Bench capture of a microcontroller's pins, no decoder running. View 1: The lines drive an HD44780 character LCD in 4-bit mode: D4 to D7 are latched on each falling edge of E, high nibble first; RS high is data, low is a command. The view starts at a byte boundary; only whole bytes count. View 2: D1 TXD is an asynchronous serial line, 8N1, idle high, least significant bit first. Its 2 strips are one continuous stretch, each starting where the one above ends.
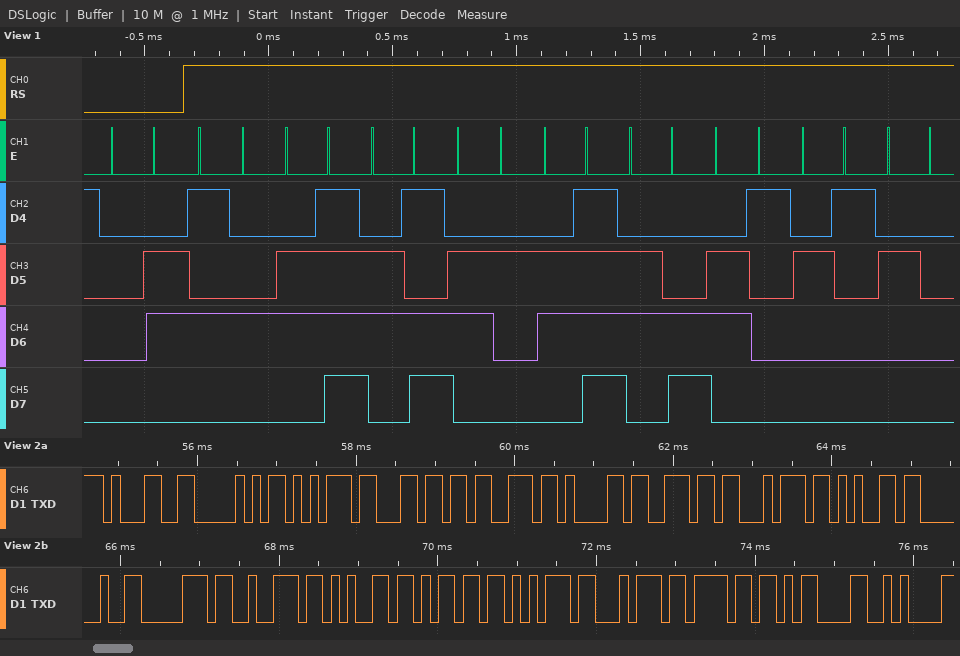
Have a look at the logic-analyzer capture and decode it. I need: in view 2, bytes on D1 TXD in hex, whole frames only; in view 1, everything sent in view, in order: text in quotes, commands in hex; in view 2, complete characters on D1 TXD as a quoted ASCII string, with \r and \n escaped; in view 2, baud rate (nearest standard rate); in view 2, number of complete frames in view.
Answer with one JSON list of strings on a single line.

["0x31 0x50 0x75 0x6C 0x73 0x61 0x6E 0x74 0x65 0x20 0x70 0x72 0x65 0x6D 0x75 0x74 0x6F 0x0D 0x0A", "0x06 \"Tombola! \"", "\"1Pulsante premuto\\r\\n\"", "9600 baud", "19"]
